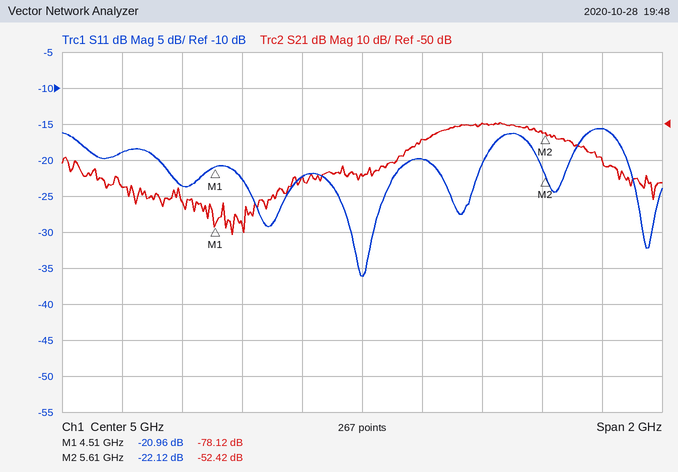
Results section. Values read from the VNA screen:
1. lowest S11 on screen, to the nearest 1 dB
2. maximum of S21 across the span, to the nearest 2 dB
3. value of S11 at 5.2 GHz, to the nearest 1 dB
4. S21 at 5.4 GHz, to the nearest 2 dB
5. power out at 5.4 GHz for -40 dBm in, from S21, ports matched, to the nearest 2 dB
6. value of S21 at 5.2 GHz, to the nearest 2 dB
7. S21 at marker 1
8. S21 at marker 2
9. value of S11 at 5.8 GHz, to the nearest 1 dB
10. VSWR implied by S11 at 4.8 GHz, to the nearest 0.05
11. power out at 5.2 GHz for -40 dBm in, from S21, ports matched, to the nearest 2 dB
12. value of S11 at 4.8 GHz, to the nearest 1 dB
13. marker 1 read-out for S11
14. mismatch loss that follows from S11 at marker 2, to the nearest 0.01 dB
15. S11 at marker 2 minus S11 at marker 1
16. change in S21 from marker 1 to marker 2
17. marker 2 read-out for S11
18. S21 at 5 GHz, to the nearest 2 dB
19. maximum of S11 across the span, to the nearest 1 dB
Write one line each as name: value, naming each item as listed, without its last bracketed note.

lowest S11 on screen, to the nearest 1 dB: -36 dB
maximum of S21 across the span, to the nearest 2 dB: -50 dB
value of S11 at 5.2 GHz, to the nearest 1 dB: -20 dB
S21 at 5.4 GHz, to the nearest 2 dB: -50 dB
power out at 5.4 GHz for -40 dBm in, from S21, ports matched, to the nearest 2 dB: -90 dBm
value of S21 at 5.2 GHz, to the nearest 2 dB: -54 dB
S21 at marker 1: -78.12 dB
S21 at marker 2: -52.42 dB
value of S11 at 5.8 GHz, to the nearest 1 dB: -16 dB
VSWR implied by S11 at 4.8 GHz, to the nearest 0.05: 1.15
power out at 5.2 GHz for -40 dBm in, from S21, ports matched, to the nearest 2 dB: -94 dBm
value of S11 at 4.8 GHz, to the nearest 1 dB: -22 dB
marker 1 read-out for S11: -20.96 dB
mismatch loss that follows from S11 at marker 2, to the nearest 0.01 dB: 0.03 dB
S11 at marker 2 minus S11 at marker 1: -1.16 dB
change in S21 from marker 1 to marker 2: 25.70 dB
marker 2 read-out for S11: -22.12 dB
S21 at 5 GHz, to the nearest 2 dB: -64 dB
maximum of S11 across the span, to the nearest 1 dB: -16 dB
